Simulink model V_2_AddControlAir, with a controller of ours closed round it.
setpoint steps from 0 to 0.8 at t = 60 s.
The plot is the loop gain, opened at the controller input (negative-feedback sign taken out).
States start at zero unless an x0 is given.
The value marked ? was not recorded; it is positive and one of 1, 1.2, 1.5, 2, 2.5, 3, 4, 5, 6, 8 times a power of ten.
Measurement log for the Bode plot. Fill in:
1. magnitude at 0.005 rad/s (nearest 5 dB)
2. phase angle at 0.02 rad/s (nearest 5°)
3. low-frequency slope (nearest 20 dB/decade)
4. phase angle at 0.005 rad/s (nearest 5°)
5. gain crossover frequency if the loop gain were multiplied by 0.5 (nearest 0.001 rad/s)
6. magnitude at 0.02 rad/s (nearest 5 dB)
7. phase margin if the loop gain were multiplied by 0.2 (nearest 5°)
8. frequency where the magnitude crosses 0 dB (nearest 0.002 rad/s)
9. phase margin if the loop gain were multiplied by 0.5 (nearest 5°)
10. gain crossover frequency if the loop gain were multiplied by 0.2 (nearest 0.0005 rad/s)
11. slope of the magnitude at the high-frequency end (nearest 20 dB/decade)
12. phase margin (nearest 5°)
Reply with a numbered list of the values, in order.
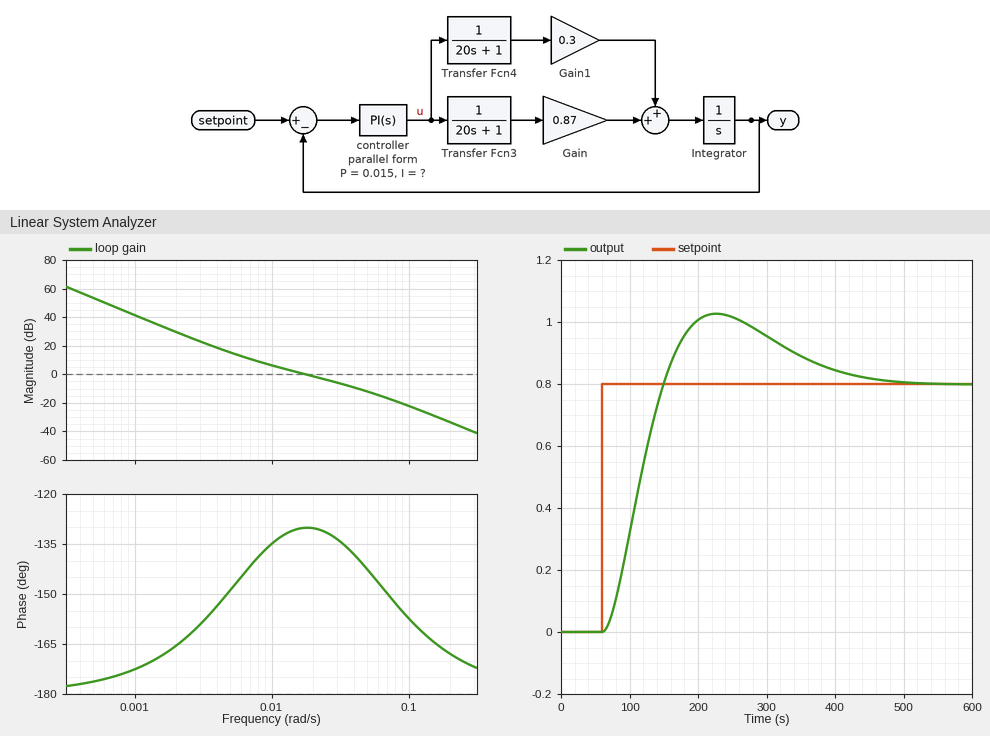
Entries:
1. 15 dB
2. -130°
3. -40 dB/decade
4. -150°
5. 0.010 rad/s
6. 0 dB
7. 35°
8. 0.018 rad/s
9. 45°
10. 0.0055 rad/s
11. -40 dB/decade
12. 50°
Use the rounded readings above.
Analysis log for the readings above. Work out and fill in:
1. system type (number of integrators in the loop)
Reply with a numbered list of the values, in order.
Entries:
1. 2
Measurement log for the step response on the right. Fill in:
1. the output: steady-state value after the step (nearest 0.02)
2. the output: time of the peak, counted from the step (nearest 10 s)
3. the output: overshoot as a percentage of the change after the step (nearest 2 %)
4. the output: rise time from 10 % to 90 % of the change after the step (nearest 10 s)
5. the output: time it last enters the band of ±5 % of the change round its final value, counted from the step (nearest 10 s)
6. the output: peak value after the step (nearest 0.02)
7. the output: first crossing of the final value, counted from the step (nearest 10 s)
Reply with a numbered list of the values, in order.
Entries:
1. 0.80
2. 170 s
3. 28 %
4. 60 s
5. 350 s
6. 1.02
7. 90 s
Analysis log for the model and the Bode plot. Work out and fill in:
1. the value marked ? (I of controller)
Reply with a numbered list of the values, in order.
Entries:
1. 0.0001
